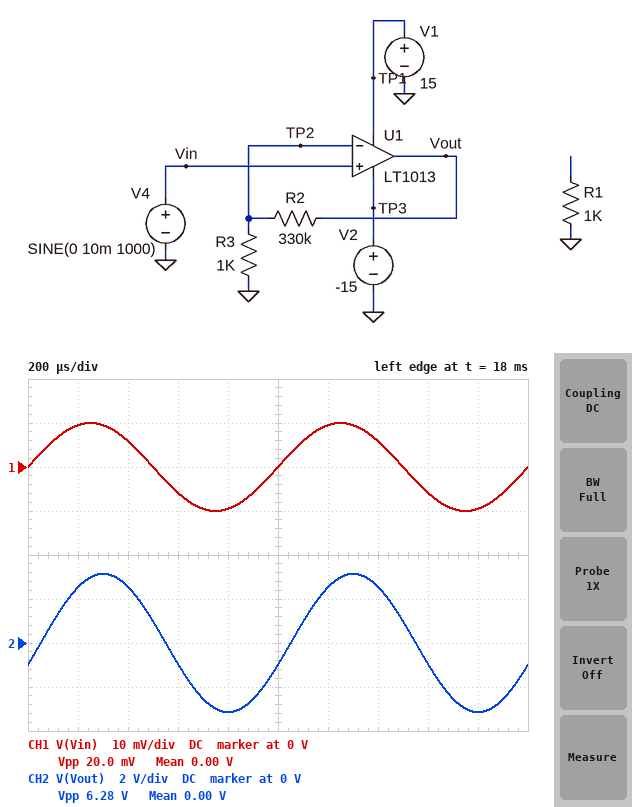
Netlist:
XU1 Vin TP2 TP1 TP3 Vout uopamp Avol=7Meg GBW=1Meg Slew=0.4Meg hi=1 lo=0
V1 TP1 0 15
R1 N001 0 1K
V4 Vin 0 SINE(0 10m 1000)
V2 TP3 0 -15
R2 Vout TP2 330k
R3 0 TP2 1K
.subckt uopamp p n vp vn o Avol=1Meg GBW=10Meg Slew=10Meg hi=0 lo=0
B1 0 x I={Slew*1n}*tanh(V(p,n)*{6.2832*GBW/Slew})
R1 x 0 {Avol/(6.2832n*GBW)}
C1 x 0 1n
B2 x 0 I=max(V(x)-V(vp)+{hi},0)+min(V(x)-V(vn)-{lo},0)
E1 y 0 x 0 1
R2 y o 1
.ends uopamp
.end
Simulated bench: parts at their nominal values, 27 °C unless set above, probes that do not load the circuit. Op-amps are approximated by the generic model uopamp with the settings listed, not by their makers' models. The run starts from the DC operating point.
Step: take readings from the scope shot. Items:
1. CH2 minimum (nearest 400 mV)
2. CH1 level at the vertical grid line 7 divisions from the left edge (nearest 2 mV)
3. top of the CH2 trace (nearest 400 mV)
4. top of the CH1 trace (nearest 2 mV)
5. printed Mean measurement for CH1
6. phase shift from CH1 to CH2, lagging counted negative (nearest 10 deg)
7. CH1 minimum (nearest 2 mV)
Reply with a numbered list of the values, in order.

1. -3.2 V
2. 6 mV
3. 3.2 V
4. 10 mV
5. 0.00 V
6. -20 deg
7. -10 mV
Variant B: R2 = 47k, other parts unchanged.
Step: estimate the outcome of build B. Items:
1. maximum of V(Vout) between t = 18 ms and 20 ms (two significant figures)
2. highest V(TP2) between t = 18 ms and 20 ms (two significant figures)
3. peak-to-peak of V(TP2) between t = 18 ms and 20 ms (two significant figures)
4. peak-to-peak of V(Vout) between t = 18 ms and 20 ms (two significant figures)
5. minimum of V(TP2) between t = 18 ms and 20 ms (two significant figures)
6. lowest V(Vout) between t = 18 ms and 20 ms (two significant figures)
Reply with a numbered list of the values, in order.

1. 480 mV
2. 10 mV
3. 20 mV
4. 960 mV
5. -10 mV
6. -480 mV
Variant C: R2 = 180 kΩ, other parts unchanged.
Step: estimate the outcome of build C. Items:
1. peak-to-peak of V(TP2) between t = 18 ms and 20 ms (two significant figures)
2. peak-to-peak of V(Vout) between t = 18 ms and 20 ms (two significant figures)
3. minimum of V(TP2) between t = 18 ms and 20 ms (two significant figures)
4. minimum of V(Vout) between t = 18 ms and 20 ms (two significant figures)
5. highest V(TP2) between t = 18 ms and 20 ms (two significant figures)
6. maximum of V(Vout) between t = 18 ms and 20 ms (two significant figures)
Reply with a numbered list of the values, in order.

1. 20 mV
2. 3.6 V
3. -9.8 mV
4. -1.8 V
5. 9.8 mV
6. 1.8 V
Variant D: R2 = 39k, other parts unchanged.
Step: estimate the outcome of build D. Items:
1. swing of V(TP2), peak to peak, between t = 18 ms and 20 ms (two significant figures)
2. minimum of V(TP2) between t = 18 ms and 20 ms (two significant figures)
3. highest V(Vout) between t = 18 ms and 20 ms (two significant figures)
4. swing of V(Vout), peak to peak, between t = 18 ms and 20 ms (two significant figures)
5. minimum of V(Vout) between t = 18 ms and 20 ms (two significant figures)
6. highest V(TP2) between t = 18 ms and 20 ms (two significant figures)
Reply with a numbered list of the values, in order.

1. 20 mV
2. -10 mV
3. 400 mV
4. 800 mV
5. -400 mV
6. 10 mV
